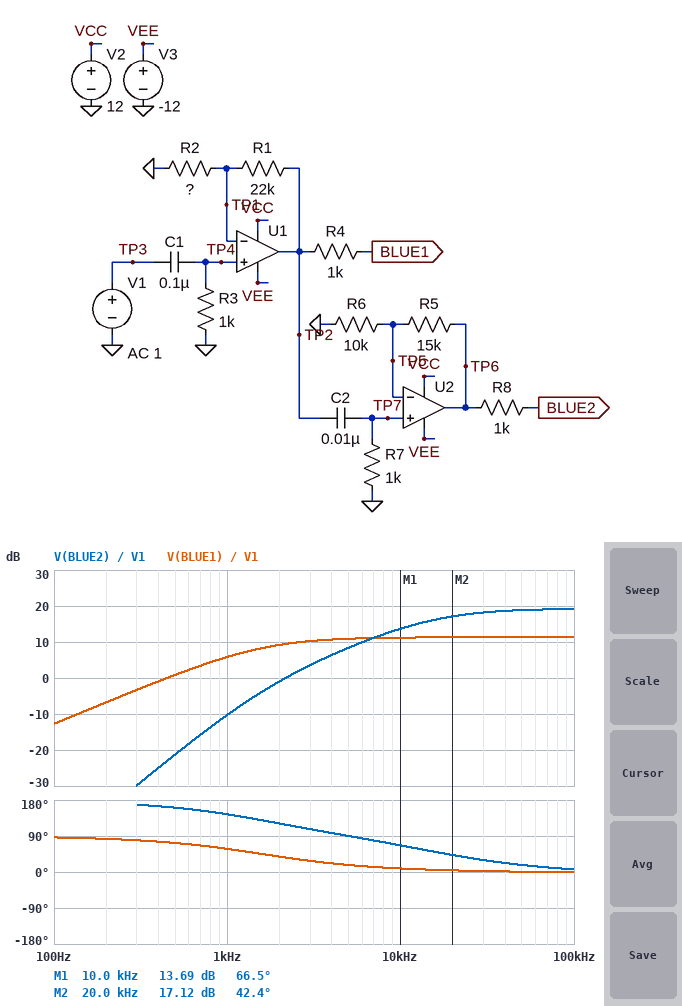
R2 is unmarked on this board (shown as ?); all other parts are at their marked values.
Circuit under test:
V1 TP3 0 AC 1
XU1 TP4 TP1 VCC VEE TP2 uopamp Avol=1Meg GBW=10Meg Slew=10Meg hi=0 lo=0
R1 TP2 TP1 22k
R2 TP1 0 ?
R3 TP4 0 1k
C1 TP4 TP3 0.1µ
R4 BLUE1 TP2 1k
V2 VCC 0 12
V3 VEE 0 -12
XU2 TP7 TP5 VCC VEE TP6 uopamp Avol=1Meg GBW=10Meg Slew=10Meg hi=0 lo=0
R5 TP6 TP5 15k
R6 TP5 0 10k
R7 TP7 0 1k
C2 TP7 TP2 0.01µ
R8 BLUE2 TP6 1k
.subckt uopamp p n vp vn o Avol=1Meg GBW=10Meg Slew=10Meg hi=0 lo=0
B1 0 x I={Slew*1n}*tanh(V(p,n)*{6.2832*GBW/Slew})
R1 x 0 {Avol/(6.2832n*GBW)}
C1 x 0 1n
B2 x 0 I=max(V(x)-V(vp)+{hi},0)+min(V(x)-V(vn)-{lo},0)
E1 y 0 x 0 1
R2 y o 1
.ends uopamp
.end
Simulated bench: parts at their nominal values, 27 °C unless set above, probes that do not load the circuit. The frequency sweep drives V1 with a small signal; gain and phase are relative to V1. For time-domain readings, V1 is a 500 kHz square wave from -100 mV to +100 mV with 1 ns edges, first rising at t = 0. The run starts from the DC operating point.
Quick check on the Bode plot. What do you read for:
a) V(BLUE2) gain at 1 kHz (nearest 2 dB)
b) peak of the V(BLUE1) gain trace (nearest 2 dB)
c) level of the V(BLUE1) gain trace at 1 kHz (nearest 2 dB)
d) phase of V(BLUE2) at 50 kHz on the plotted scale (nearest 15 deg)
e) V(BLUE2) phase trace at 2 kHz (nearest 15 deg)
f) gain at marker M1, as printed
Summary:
-10 dB
12 dB
6 dB
15 deg
120 deg
13.69 dB
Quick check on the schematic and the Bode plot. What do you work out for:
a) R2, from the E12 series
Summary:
8.2 kΩ
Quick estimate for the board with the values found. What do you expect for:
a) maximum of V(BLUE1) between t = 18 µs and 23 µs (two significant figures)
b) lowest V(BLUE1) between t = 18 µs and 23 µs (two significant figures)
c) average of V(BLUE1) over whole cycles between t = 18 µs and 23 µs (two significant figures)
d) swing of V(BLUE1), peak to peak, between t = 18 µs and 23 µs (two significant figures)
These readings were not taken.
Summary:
670 mV
-73 mV
300 mV
750 mV
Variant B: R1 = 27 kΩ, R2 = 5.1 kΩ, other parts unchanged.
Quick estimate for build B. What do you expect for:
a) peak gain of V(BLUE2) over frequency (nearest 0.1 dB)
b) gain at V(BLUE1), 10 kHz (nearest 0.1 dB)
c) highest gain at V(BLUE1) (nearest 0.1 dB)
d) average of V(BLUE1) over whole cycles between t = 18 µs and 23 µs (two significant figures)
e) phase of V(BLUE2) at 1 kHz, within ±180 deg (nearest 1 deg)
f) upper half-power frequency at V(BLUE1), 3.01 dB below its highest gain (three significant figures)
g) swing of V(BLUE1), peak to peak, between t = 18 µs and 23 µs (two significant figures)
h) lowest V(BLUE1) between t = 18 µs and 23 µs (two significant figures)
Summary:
23.8 dB
15.9 dB
16.0 dB
510 mV
144 deg
1.59 MHz
1.3 V
-120 mV
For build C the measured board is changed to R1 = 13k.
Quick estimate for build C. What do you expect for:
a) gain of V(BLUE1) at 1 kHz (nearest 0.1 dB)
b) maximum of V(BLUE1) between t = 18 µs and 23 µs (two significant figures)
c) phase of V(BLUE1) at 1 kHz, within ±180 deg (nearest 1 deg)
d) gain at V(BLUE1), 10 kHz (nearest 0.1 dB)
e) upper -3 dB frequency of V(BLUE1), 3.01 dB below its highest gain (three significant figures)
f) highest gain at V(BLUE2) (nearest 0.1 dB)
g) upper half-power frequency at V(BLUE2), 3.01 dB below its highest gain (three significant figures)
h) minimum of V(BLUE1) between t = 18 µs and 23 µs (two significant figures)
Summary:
2.8 dB
470 mV
58 deg
8.1 dB
3.87 MHz
16.2 dB
2.55 MHz
-51 mV
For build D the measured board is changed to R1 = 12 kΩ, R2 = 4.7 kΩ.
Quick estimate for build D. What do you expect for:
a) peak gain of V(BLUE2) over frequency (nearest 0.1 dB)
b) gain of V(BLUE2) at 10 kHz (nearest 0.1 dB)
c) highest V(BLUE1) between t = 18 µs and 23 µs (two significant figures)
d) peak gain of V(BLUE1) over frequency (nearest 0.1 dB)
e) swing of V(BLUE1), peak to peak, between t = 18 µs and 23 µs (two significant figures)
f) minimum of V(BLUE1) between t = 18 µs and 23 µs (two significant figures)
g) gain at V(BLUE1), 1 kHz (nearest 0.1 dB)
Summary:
18.9 dB
13.4 dB
650 mV
11.0 dB
720 mV
-70 mV
5.5 dB
